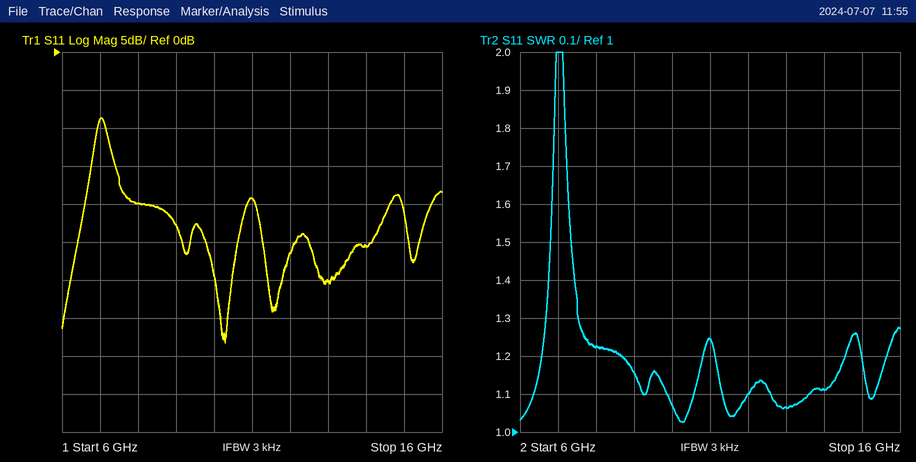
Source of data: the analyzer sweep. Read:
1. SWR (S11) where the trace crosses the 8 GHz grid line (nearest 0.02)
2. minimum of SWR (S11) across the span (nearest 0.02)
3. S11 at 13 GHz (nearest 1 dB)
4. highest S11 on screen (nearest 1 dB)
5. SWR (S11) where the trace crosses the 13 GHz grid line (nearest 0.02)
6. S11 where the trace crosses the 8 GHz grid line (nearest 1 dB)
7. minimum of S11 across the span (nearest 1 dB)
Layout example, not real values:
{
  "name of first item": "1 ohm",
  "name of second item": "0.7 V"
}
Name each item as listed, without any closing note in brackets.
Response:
{
  "SWR (S11) where the trace crosses the 8 GHz grid line": "1.22",
  "minimum of SWR (S11) across the span": "1.02",
  "S11 at 13 GHz": "-30 dB",
  "highest S11 on screen": "-9 dB",
  "SWR (S11) where the trace crosses the 13 GHz grid line": "1.06",
  "S11 where the trace crosses the 8 GHz grid line": "-20 dB",
  "minimum of S11 across the span": "-38 dB"
}
